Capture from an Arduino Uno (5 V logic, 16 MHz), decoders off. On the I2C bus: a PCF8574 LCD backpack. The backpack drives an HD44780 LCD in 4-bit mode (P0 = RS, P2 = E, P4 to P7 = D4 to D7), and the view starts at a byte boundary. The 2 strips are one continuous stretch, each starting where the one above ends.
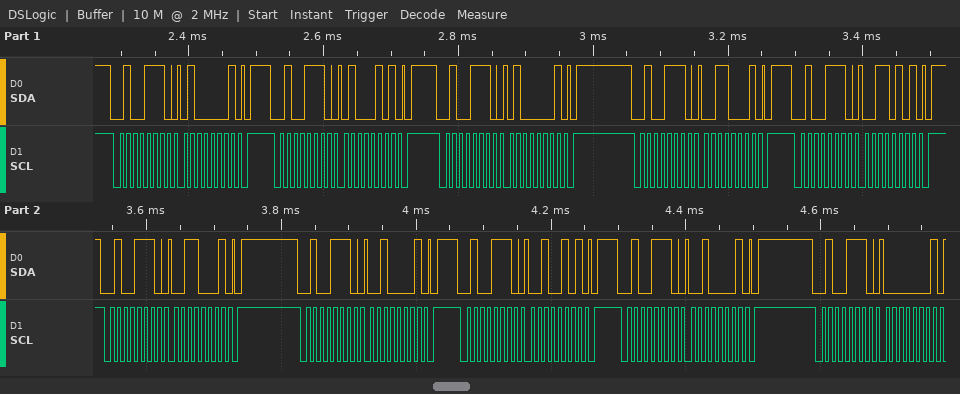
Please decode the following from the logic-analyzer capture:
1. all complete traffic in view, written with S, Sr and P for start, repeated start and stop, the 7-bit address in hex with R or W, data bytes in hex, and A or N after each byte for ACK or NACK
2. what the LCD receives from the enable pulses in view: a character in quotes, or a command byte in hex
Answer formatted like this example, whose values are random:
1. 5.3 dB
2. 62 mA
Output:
1. S 27W A 41 A P S 27W A 45 A P S 27W A 41 A P S 27W A 31 A P S 27W A 35 A P S 27W A 31 A P S 27W A 21 A P S 27W A 25 A P S 27W A 21 A P S 27W A 01 A
2. 'C'
